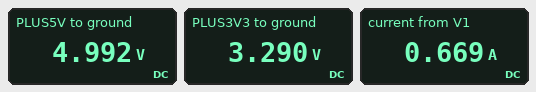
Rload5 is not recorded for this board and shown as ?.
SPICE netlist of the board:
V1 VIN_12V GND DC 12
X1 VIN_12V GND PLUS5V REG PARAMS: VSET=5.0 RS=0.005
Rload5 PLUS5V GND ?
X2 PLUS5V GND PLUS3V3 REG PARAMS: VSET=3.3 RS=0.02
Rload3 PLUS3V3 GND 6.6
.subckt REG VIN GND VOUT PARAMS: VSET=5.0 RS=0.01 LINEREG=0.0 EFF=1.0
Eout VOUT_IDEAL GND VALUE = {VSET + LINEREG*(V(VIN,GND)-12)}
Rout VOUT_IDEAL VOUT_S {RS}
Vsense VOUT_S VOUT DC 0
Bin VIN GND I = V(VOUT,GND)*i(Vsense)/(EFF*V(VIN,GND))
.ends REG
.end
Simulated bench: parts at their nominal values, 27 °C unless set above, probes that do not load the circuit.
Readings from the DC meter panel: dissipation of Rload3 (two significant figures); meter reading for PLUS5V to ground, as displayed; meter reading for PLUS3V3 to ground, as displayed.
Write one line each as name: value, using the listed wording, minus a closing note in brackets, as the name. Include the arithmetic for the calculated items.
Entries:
dissipation of Rload3: (3.29 V)^2 / 6.6 Ω = 1.6 W
meter reading for PLUS5V to ground, as displayed: 4.992 V
meter reading for PLUS3V3 to ground, as displayed: 3.290 V
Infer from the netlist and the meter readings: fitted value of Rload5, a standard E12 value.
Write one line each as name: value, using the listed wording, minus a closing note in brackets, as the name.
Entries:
fitted value of Rload5, a standard E12 value: 3.9 Ω
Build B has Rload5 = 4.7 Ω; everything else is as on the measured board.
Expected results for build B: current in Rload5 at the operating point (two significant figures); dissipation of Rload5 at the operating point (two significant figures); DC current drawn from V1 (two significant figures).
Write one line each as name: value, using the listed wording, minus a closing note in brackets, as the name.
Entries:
current in Rload5 at the operating point: 1.1 A
dissipation of Rload5 at the operating point: 5.3 W
DC current drawn from V1: 580 mA
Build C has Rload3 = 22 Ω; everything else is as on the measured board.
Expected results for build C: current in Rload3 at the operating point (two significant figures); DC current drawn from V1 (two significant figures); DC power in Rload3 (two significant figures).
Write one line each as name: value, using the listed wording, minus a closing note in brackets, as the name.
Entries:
current in Rload3 at the operating point: 150 mA
DC current drawn from V1: 570 mA
DC power in Rload3: 490 mW
